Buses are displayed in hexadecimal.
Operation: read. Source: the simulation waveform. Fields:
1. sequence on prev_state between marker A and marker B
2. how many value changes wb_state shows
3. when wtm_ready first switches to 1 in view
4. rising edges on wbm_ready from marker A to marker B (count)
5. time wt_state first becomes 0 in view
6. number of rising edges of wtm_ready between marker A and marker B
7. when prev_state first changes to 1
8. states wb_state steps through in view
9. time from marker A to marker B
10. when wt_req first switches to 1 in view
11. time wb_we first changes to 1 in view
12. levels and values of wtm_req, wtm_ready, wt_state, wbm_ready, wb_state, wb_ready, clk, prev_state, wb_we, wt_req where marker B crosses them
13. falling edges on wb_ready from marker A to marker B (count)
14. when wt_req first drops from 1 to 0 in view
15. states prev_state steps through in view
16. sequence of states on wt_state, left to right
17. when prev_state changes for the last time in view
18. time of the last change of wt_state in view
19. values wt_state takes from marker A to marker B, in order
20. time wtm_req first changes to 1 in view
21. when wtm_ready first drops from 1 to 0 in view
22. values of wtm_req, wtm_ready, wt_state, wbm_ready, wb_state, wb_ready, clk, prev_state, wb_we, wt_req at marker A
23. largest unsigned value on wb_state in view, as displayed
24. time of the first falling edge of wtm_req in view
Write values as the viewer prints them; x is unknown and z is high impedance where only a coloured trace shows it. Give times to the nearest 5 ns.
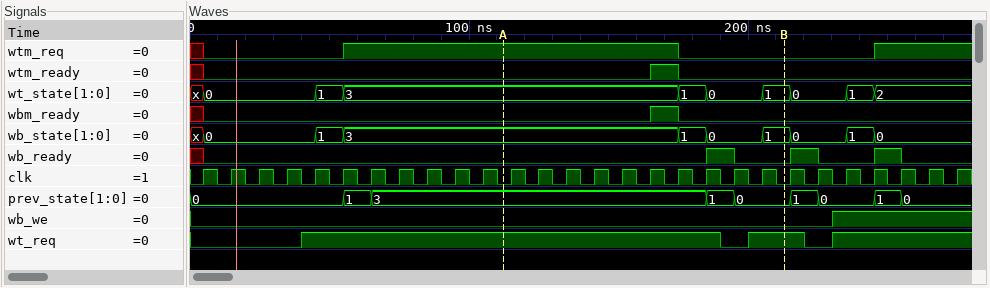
3, 1, 0
9
165 ns
1
5 ns
1
55 ns
x, 0, 1, 3, 1, 0, 1, 0, 1, 0
100 ns
40 ns
230 ns
wtm_req=0, wtm_ready=0, wt_state=1, wbm_ready=0, wb_state=1, wb_ready=0, clk=0, prev_state=0, wb_we=0, wt_req=1
1
190 ns
0, 1, 3, 1, 0, 1, 0, 1, 0
x, 0, 1, 3, 1, 0, 1, 0, 1, 2
255 ns
245 ns
3, 1, 0, 1
55 ns
175 ns
wtm_req=1, wtm_ready=0, wt_state=3, wbm_ready=0, wb_state=3, wb_ready=0, clk=0, prev_state=3, wb_we=0, wt_req=1
3
175 ns
